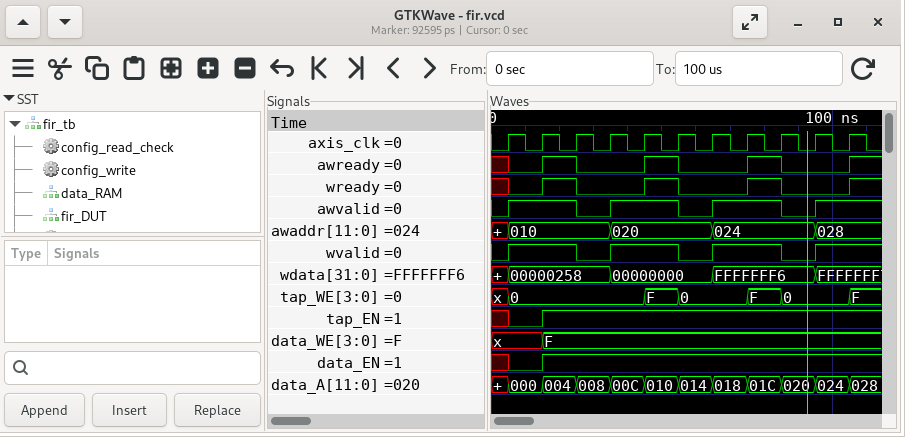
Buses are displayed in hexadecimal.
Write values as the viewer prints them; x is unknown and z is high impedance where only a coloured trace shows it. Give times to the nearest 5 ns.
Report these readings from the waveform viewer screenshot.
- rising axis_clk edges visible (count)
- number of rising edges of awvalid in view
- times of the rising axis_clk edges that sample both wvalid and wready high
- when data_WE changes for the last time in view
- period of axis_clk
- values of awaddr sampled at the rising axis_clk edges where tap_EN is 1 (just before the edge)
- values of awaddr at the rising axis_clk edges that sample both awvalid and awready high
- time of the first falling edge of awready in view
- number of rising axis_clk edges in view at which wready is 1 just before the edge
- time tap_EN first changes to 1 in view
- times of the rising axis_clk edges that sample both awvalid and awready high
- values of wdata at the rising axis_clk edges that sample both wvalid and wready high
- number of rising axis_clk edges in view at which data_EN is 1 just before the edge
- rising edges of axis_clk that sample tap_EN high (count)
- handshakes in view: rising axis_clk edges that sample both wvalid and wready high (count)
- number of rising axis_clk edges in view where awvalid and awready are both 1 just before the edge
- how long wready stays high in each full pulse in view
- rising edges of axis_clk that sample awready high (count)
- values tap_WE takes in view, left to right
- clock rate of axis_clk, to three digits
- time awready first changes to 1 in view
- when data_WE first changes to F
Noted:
11
4
25 ns, 55 ns, 85 ns
15 ns
10 ns
010, 010, 020, 020, 020, 024, 024, 024, 028
010, 020, 024
25 ns
3
15 ns
25 ns, 55 ns, 85 ns
00000258, 00000000, FFFFFFF6
9
9
3
3
10 ns, 10 ns, 10 ns
3
x, 0, F, 0, F, 0, F
100 MHz
15 ns
15 ns
